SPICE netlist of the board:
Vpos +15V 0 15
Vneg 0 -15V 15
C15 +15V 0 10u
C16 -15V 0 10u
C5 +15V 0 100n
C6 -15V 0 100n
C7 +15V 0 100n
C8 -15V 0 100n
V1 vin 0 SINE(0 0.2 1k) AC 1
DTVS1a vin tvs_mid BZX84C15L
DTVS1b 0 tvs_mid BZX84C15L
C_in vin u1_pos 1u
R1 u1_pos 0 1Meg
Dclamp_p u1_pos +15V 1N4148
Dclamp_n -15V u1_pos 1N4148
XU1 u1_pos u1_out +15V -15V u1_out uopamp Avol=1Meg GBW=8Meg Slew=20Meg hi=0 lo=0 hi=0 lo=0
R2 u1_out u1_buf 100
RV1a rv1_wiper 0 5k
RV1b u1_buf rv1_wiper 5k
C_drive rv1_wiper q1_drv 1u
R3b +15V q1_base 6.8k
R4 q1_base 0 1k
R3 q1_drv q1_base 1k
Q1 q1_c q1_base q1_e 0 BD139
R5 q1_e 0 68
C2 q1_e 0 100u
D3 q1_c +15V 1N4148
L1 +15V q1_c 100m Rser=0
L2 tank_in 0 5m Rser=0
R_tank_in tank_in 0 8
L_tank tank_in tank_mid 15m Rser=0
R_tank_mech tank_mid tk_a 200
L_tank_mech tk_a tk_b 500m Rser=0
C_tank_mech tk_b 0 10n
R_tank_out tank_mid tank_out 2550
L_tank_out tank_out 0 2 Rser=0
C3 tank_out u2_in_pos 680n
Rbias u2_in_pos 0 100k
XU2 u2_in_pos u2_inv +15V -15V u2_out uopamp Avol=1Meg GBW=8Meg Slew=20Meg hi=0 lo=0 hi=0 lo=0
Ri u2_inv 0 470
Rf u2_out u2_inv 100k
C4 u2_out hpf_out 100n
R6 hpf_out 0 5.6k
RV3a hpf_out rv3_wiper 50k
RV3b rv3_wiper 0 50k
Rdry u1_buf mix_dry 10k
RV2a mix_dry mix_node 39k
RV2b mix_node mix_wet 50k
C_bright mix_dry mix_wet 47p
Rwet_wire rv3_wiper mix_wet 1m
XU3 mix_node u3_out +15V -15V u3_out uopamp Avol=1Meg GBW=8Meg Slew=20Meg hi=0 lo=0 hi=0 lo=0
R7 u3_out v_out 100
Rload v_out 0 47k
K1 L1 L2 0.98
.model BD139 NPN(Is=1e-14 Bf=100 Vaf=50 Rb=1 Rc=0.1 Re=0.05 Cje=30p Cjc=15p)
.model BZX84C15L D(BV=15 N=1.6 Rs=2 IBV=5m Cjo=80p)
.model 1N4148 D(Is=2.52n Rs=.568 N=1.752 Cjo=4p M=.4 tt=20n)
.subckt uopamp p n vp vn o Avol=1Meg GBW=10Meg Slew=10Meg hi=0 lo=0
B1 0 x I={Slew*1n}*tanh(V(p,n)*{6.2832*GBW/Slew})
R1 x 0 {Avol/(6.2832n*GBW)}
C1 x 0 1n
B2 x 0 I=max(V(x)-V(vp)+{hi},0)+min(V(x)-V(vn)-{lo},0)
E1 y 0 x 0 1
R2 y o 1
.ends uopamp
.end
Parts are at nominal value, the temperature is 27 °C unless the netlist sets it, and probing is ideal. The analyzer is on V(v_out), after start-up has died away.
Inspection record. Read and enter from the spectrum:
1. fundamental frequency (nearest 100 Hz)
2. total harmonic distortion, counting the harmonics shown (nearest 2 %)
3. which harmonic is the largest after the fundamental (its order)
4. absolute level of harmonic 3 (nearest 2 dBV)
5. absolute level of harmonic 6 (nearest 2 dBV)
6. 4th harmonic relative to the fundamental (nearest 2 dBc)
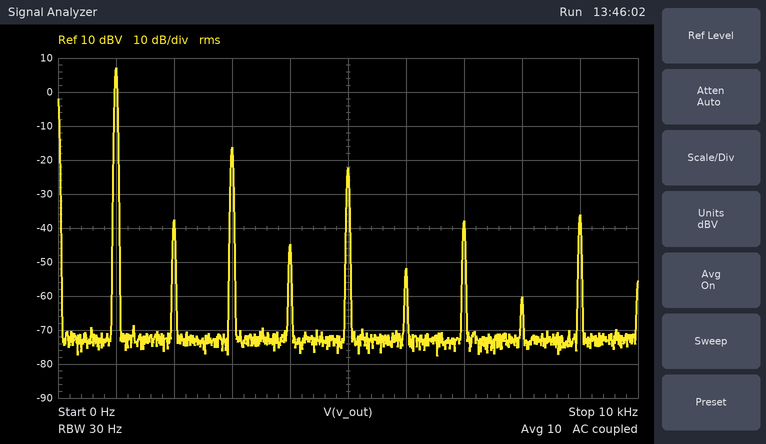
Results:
1.0 kHz
8 %
3
-16 dBV
-52 dBV
-52 dBc
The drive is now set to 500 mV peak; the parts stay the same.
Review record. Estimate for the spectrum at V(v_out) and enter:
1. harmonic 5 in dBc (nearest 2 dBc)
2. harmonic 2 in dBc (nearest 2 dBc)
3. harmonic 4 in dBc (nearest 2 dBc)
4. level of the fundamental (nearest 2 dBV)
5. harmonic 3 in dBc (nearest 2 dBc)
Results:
-20 dBc
-18 dBc
-20 dBc
8 dBV
-12 dBc
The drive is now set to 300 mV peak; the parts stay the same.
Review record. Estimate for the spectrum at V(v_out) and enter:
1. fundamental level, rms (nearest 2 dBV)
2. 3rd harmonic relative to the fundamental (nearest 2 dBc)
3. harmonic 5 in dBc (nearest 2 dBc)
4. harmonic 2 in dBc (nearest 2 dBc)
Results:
8 dBV
-14 dBc
-32 dBc
-32 dBc
